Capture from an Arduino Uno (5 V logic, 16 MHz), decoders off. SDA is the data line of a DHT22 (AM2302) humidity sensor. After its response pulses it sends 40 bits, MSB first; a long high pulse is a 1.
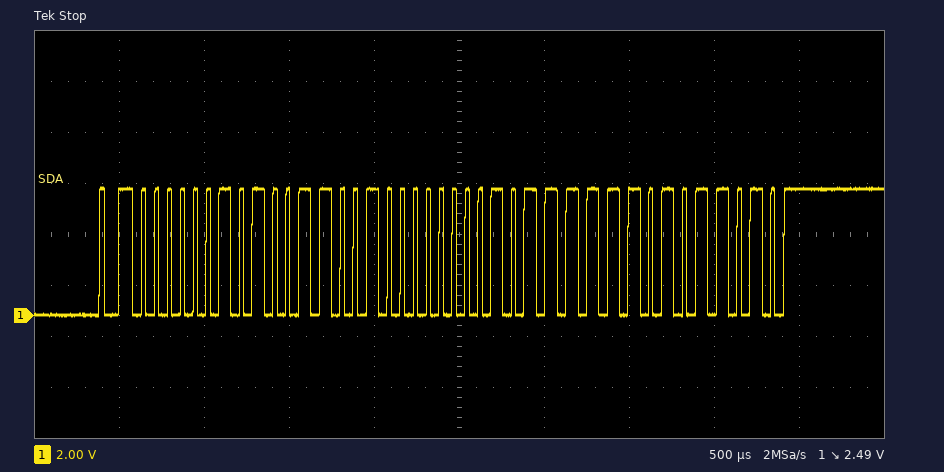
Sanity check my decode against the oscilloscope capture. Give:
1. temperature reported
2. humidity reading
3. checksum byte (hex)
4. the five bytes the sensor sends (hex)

19.1 °C
66.5 %
0x5A
02 99 00 BF 5A
